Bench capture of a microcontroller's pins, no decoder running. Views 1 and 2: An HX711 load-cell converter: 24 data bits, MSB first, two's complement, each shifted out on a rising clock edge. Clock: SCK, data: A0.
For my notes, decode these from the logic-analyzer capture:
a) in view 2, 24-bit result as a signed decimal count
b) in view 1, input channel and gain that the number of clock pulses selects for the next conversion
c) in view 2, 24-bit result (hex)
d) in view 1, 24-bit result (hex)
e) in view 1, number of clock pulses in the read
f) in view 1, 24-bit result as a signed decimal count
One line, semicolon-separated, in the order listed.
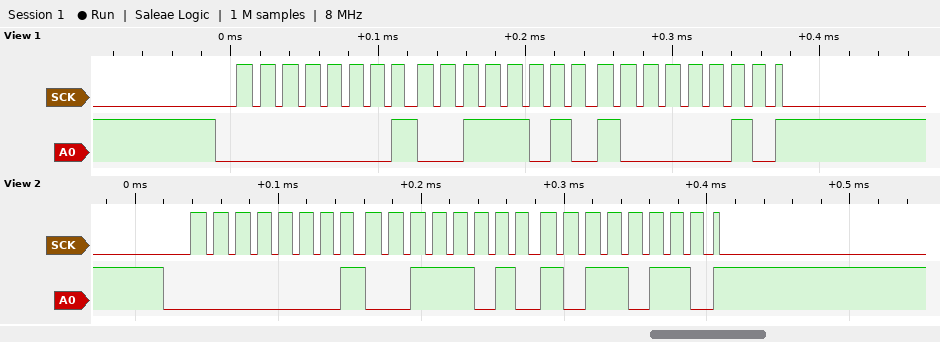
80566; channel A, gain 128; 0x013AB6; 0x013A82; 25; 80514
